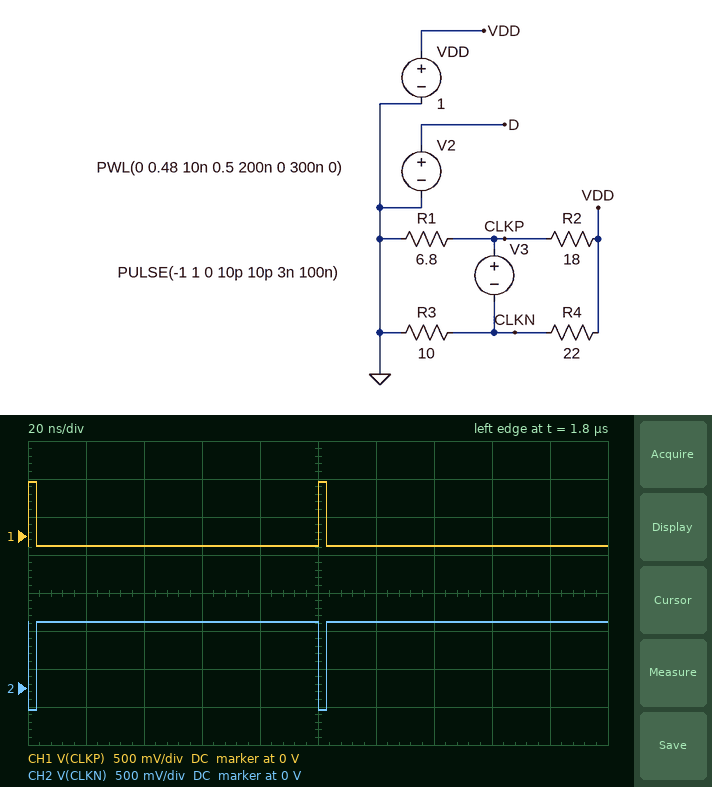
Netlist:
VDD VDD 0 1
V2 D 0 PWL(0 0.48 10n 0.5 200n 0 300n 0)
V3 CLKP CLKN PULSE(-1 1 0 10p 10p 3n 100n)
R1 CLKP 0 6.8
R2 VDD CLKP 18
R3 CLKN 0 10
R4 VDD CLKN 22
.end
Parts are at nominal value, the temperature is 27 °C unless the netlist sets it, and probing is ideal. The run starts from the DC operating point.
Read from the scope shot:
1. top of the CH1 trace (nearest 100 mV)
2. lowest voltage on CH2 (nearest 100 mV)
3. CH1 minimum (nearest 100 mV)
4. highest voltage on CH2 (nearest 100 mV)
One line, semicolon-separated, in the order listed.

700 mV; -300 mV; -100 mV; 900 mV
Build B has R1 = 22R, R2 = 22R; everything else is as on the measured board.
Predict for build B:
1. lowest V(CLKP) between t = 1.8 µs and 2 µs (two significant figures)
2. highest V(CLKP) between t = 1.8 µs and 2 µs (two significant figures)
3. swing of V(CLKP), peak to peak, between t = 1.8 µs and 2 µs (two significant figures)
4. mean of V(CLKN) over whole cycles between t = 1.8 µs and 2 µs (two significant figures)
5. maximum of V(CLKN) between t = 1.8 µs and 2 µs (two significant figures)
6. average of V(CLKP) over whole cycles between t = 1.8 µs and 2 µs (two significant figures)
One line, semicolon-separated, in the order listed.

-230 mV; 1.0 V; 1.2 V; 750 mV; 770 mV; -190 mV
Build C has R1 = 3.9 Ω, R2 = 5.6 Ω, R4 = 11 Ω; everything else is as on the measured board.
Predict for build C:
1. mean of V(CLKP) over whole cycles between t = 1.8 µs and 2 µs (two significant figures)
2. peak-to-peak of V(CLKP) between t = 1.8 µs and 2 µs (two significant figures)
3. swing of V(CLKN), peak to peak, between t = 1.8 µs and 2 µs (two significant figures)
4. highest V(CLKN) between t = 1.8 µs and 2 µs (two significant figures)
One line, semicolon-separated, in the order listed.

140 mV; 610 mV; 1.4 V; 1.1 V
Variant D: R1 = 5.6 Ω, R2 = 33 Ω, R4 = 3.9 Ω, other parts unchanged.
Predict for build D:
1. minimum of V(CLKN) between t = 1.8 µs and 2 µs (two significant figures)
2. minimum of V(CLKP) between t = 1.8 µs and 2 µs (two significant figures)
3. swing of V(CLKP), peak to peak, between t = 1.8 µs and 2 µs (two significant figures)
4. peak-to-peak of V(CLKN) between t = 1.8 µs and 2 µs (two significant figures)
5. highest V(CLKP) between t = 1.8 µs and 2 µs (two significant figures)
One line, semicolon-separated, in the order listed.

140 mV; -120 mV; 1.3 V; 740 mV; 1.1 V
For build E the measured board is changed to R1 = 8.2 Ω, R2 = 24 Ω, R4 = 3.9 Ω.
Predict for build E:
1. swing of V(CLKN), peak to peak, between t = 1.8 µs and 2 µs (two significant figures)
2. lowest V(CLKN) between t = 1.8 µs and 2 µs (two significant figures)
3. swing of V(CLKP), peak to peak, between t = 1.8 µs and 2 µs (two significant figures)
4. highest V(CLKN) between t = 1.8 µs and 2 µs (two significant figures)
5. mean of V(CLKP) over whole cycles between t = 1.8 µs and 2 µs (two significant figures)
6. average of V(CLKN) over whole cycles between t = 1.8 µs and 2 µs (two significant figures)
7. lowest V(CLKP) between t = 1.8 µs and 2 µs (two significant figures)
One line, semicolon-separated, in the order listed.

630 mV; 260 mV; 1.4 V; 890 mV; -71 mV; 870 mV; -110 mV
